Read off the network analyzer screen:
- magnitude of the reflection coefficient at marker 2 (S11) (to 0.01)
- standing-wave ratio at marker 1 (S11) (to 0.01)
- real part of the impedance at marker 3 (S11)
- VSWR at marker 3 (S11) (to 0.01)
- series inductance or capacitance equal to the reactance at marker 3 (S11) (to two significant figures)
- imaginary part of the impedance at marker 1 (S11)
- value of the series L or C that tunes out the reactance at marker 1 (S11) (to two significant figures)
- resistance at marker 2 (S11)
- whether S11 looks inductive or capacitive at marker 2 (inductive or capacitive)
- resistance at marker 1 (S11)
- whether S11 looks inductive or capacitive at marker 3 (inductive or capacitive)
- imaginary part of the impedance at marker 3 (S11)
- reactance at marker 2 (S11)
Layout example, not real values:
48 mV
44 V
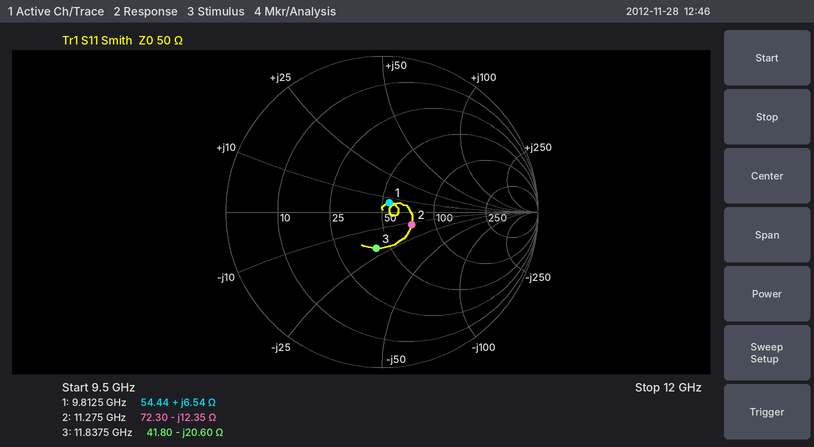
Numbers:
0.21
1.16
41.80 Ω
1.62
650 fF
+6.54 Ω
2.5 pF
72.30 Ω
capacitive
54.44 Ω
capacitive
-20.60 Ω
-12.35 Ω
